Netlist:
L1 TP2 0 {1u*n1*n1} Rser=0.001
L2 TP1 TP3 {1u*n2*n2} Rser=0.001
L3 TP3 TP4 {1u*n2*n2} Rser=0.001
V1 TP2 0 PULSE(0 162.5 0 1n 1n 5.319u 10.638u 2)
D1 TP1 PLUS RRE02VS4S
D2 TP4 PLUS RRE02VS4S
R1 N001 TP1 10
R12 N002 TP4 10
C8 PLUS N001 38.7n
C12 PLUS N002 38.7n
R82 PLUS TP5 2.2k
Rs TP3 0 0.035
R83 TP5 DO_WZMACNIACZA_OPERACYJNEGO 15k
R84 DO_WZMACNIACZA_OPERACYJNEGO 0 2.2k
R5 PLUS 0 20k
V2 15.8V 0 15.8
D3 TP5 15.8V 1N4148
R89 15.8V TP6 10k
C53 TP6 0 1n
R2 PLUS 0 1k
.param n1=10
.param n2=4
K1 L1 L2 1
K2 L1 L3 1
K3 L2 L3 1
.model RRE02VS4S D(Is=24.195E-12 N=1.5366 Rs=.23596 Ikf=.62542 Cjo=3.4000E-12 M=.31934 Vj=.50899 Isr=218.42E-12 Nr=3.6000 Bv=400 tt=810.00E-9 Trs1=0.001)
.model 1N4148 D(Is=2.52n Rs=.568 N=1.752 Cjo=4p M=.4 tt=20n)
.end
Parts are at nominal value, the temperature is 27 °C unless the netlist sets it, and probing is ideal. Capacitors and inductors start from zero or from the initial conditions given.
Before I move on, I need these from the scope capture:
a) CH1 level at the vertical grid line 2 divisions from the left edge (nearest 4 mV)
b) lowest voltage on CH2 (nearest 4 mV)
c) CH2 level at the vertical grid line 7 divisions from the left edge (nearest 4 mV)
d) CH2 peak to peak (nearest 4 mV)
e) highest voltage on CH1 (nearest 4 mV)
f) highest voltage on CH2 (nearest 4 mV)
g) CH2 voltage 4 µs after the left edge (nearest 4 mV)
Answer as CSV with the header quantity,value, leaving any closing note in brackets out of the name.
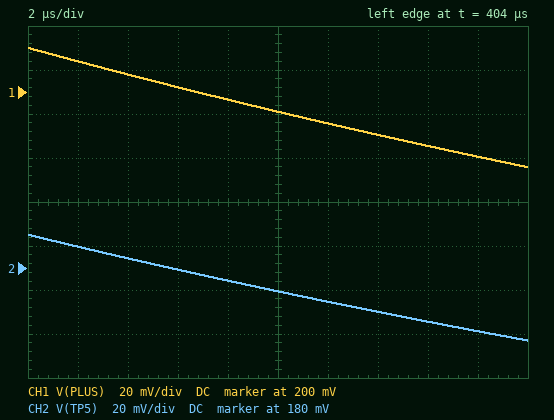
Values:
quantity,value
CH1 level at the vertical grid line 2 divisions from the left edge,208 mV
lowest voltage on CH2,148 mV
CH2 level at the vertical grid line 7 divisions from the left edge,160 mV
CH2 peak to peak,48 mV
highest voltage on CH1,220 mV
highest voltage on CH2,196 mV
CH2 voltage 4 µs after the left edge,184 mV
